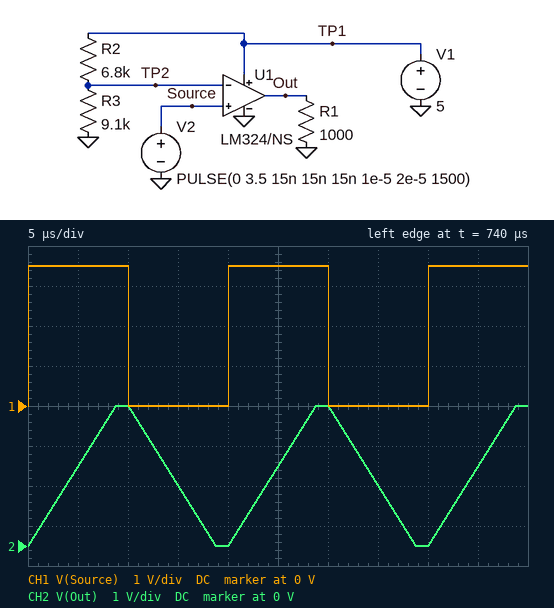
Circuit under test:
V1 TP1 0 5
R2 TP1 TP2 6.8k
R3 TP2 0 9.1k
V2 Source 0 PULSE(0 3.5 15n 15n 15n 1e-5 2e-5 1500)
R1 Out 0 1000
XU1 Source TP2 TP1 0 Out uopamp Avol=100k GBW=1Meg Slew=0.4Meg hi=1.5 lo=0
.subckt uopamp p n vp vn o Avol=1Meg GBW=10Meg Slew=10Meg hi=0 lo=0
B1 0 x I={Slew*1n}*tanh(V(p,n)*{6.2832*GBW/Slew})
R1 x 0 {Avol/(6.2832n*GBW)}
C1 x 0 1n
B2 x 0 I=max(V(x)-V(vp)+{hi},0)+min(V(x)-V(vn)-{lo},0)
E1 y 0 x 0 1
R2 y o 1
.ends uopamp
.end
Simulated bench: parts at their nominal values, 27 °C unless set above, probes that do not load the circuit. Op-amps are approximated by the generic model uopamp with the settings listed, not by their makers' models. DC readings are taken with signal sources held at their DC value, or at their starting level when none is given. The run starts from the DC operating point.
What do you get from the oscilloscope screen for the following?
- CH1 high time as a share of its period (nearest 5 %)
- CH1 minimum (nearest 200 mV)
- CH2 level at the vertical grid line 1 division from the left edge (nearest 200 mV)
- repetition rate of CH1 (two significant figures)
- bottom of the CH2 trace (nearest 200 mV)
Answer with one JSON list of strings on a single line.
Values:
["50 %", "0 V", "2.0 V", "50 kHz", "0 V"]
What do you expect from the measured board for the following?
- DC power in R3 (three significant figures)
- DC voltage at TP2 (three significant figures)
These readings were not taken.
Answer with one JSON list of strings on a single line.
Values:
["900 µW", "2.86 V"]
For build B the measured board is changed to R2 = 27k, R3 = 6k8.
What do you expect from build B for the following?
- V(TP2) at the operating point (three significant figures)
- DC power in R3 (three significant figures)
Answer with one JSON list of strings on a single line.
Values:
["1.01 V", "149 µW"]
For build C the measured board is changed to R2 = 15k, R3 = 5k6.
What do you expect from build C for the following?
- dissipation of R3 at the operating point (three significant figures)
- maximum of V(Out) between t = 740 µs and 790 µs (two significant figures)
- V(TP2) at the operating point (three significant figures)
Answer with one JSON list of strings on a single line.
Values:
["330 µW", "3.5 V", "1.36 V"]
